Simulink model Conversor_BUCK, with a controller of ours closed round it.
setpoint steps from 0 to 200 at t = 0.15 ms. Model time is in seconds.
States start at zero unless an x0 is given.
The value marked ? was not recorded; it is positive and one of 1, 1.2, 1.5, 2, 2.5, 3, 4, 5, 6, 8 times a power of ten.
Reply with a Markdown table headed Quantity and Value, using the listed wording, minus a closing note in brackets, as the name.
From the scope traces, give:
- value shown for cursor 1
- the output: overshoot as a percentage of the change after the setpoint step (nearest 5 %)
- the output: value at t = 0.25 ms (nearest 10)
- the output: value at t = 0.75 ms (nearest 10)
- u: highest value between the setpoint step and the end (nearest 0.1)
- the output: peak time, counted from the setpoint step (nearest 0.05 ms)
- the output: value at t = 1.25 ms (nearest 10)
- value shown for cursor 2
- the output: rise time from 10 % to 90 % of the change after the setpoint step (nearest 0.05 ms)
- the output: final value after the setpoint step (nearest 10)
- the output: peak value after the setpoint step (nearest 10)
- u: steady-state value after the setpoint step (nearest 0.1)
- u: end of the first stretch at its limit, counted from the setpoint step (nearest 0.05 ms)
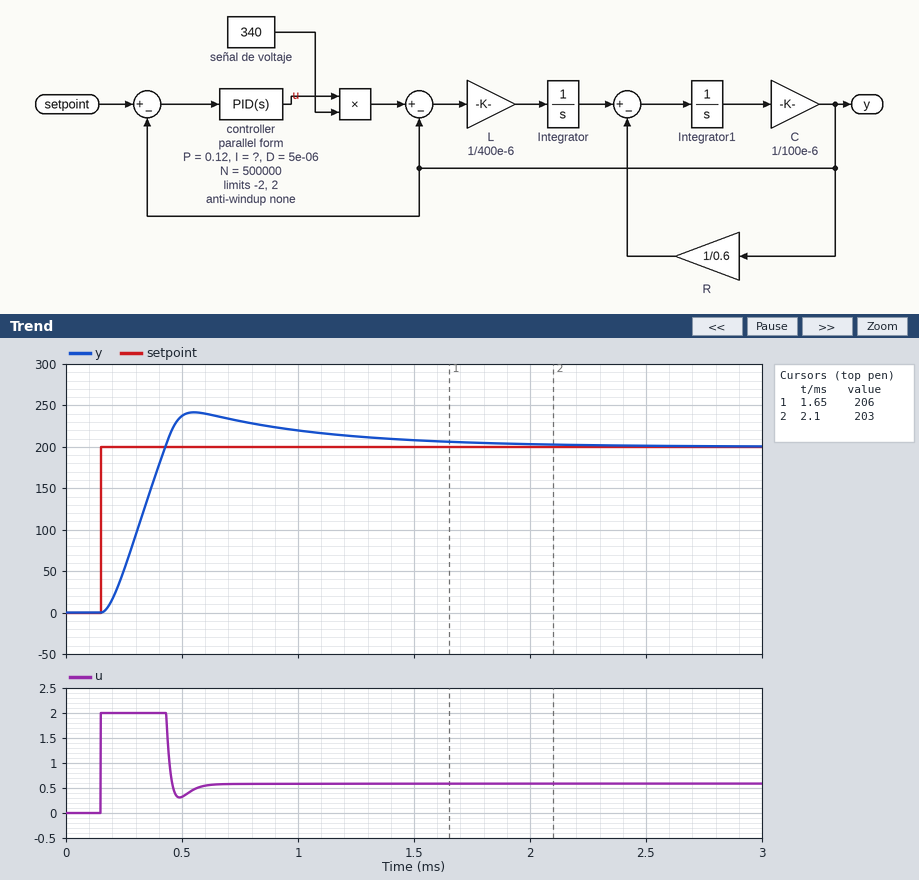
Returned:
| Quantity | Value |
|---|---|
| value shown for cursor 1 | 206 |
| the output: overshoot as a percentage of the change after the setpoint step | 20 % |
| the output: value at t = 0.25 ms | 50 |
| the output: value at t = 0.75 ms | 230 |
| u: highest value between the setpoint step and the end | 2.0 |
| the output: peak time, counted from the setpoint step | 0.40 ms |
| the output: value at t = 1.25 ms | 210 |
| value shown for cursor 2 | 203 |
| the output: rise time from 10 % to 90 % of the change after the setpoint step | 0.20 ms |
| the output: final value after the setpoint step | 200 |
| the output: peak value after the setpoint step | 240 |
| u: steady-state value after the setpoint step | 0.6 |
| u: end of the first stretch at its limit, counted from the setpoint step | 0.30 ms |
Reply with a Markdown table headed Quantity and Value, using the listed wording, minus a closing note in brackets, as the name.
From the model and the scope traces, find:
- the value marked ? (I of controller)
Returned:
| Quantity | Value |
|---|---|
| the value marked ? | 200 |
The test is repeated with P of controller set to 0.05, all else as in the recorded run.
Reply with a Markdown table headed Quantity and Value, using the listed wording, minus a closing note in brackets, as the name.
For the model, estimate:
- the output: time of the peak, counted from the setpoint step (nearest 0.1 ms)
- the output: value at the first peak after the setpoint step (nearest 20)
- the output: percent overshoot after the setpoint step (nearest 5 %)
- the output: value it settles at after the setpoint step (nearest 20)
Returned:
| Quantity | Value |
|---|---|
| the output: time of the peak, counted from the setpoint step | 0.5 ms |
| the output: value at the first peak after the setpoint step | 280 |
| the output: percent overshoot after the setpoint step | 35 % |
| the output: value it settles at after the setpoint step | 200 |
